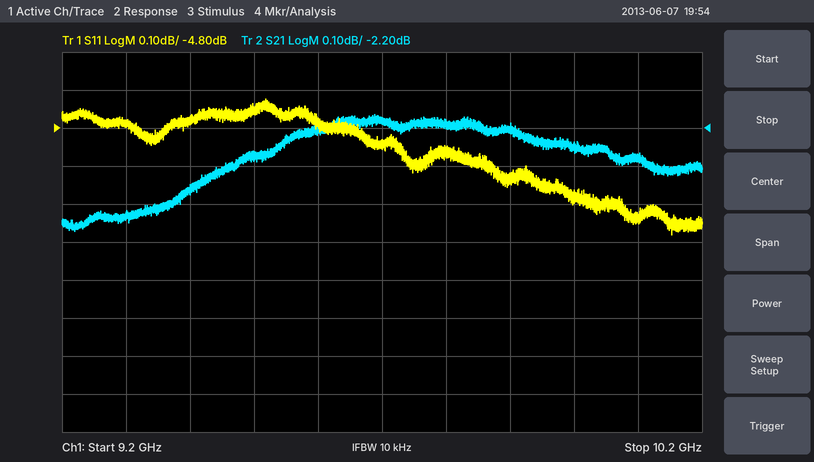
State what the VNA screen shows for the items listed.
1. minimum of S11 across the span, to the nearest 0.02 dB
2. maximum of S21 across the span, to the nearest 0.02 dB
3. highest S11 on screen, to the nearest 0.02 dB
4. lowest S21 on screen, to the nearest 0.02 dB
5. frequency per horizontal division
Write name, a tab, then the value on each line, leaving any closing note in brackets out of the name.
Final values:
minimum of S11 across the span, to the nearest 0.02 dB	-5.08 dB
maximum of S21 across the span, to the nearest 0.02 dB	-2.16 dB
highest S11 on screen, to the nearest 0.02 dB	-4.72 dB
lowest S21 on screen, to the nearest 0.02 dB	-2.48 dB
frequency per horizontal division	100 MHz
